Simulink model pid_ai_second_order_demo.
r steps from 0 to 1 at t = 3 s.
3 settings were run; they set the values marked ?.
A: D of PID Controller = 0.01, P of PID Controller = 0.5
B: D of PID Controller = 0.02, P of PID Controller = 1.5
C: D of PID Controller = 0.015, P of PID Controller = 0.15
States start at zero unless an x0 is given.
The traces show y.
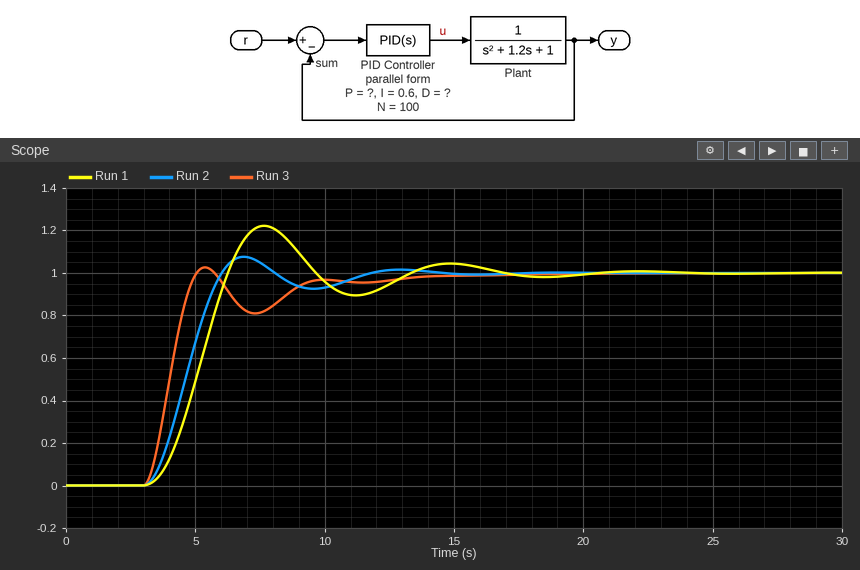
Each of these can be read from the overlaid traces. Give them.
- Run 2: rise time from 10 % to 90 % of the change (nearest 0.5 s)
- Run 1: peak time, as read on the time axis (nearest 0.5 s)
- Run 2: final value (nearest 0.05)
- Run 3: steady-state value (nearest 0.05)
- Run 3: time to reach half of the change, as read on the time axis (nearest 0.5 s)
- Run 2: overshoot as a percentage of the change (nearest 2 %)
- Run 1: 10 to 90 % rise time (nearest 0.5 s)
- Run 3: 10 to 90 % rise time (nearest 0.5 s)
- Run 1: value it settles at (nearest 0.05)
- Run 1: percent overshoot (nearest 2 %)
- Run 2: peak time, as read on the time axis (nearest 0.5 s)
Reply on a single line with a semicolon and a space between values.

2.0 s; 7.5 s; 1.00; 1.00; 4.0 s; 8 %; 2.0 s; 1.5 s; 1.00; 22 %; 7.0 s
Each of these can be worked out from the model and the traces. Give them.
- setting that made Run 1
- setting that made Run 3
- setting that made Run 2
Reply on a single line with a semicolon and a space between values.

C; B; A
